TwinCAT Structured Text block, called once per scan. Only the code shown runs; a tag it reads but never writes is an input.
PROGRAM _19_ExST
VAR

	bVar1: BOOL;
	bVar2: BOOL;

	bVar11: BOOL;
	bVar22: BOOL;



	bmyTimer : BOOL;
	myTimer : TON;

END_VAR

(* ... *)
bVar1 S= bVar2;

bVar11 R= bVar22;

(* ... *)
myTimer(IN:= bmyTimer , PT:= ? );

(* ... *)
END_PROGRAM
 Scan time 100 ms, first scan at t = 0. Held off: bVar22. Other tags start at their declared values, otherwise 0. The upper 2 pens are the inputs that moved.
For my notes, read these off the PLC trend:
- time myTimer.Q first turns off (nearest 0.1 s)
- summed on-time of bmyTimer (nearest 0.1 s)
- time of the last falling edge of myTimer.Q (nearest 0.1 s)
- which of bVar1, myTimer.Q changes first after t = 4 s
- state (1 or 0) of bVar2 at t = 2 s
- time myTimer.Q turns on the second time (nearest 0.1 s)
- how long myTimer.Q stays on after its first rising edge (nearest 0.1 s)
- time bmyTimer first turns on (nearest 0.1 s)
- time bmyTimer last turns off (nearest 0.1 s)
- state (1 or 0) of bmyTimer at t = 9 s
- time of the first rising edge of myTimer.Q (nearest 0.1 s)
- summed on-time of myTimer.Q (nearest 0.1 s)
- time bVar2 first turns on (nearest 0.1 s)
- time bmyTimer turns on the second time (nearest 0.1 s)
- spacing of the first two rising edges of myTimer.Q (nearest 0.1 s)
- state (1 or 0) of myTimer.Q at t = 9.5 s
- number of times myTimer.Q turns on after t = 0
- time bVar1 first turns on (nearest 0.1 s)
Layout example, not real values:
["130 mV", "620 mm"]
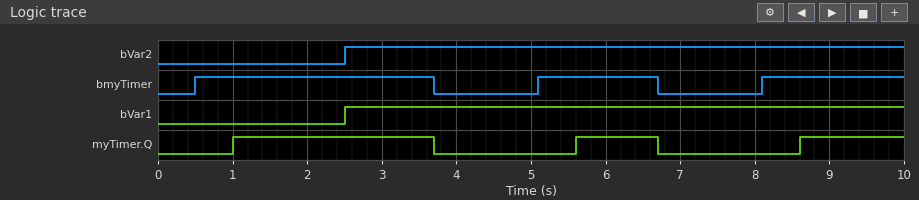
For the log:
["3.7 s", "6.7 s", "6.7 s", "myTimer.Q", "0", "5.6 s", "2.7 s", "0.5 s", "6.7 s", "1", "1.0 s", "5.2 s", "2.5 s", "5.1 s", "4.6 s", "1", "3", "2.5 s"]
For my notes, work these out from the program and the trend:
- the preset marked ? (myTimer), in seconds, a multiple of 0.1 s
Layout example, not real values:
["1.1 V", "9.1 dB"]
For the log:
["0.5 s"]
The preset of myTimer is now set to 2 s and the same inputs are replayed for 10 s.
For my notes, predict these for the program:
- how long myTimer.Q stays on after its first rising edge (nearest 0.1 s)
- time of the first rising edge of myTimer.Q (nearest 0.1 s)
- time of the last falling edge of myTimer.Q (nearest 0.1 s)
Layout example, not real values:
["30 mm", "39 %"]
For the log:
["1.2 s", "2.5 s", "3.7 s"]
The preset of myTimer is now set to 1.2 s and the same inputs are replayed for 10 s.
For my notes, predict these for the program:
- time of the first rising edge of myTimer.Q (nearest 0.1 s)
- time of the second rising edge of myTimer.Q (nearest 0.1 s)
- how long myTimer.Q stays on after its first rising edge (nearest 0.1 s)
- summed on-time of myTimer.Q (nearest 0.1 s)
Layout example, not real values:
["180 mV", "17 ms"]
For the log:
["1.7 s", "6.3 s", "2.0 s", "3.1 s"]
